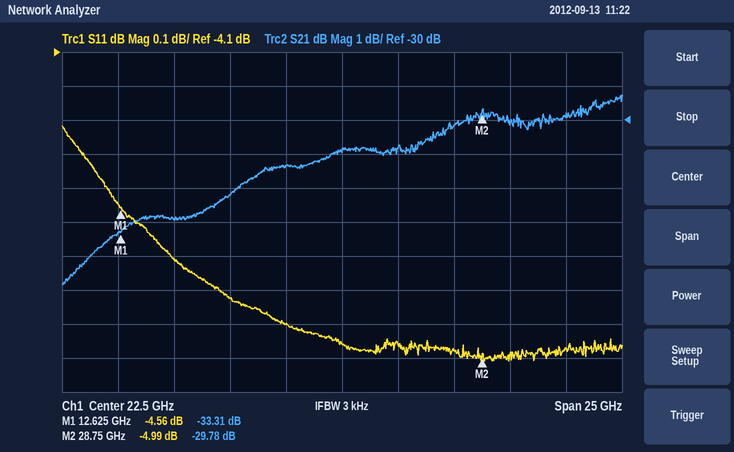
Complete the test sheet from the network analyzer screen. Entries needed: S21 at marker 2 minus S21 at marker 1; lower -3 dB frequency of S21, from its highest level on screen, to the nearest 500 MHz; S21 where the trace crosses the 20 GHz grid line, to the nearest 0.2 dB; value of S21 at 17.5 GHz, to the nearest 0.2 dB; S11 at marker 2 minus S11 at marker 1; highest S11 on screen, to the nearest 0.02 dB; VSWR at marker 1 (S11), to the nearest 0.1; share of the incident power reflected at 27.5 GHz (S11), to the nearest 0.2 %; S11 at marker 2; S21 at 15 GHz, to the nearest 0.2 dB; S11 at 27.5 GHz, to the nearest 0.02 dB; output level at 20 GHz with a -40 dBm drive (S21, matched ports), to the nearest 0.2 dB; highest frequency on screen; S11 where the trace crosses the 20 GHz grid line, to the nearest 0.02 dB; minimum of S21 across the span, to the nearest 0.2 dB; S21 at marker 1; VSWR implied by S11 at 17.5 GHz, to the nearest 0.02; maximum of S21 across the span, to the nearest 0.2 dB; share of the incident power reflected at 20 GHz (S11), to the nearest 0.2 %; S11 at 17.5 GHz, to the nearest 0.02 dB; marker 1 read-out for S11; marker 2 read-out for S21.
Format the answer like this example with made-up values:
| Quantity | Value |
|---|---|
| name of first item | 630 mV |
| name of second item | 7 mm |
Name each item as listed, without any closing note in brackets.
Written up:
| Quantity | Value |
|---|---|
| S21 at marker 2 minus S21 at marker 1 | 3.53 dB |
| lower -3 dB frequency of S21, from its highest level on screen, to the nearest 500 MHz | 17.5 GHz |
| S21 where the trace crosses the 20 GHz grid line, to the nearest 0.2 dB | -31.4 dB |
| value of S21 at 17.5 GHz, to the nearest 0.2 dB | -32.2 dB |
| S11 at marker 2 minus S11 at marker 1 | -0.43 dB |
| highest S11 on screen, to the nearest 0.02 dB | -4.32 dB |
| VSWR at marker 1 (S11), to the nearest 0.1 | 3.9 |
| share of the incident power reflected at 27.5 GHz (S11), to the nearest 0.2 % | 31.8 % |
| S11 at marker 2 | -4.99 dB |
| S21 at 15 GHz, to the nearest 0.2 dB | -33.0 dB |
| S11 at 27.5 GHz, to the nearest 0.02 dB | -4.98 dB |
| output level at 20 GHz with a -40 dBm drive (S21, matched ports), to the nearest 0.2 dB | -71.4 dBm |
| highest frequency on screen | 35 GHz |
| S11 where the trace crosses the 20 GHz grid line, to the nearest 0.02 dB | -4.90 dB |
| minimum of S21 across the span, to the nearest 0.2 dB | -34.8 dB |
| S21 at marker 1 | -33.31 dB |
| VSWR implied by S11 at 17.5 GHz, to the nearest 0.02 | 3.70 |
| maximum of S21 across the span, to the nearest 0.2 dB | -29.2 dB |
| share of the incident power reflected at 20 GHz (S11), to the nearest 0.2 % | 32.4 % |
| S11 at 17.5 GHz, to the nearest 0.02 dB | -4.82 dB |
| marker 1 read-out for S11 | -4.56 dB |
| marker 2 read-out for S21 | -29.78 dB |
